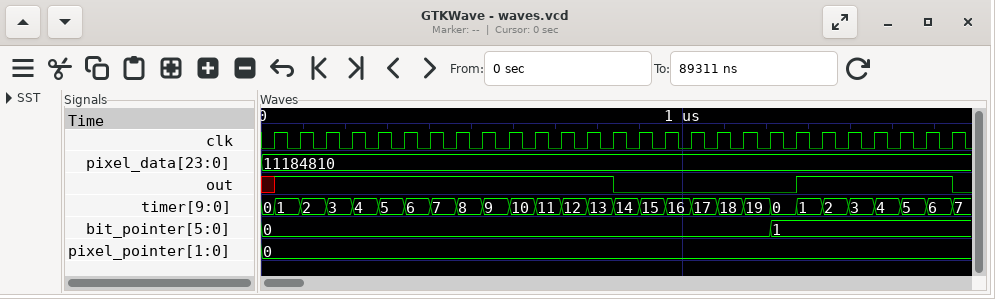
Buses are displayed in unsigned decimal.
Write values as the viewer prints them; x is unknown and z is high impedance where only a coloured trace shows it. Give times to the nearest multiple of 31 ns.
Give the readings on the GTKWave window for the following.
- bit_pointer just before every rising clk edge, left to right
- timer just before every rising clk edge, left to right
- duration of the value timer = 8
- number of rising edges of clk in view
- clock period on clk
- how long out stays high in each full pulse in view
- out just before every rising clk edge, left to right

0, 0, 0, 0, 0, 0, 0, 0, 0, 0, 0, 0, 0, 0, 0, 0, 0, 0, 0, 0, 1, 1, 1, 1, 1, 1, 1
0, 1, 2, 3, 4, 5, 6, 7, 8, 9, 10, 11, 12, 13, 14, 15, 16, 17, 18, 19, 0, 1, 2, 3, 4, 5, 6
62 ns
27
62 ns
372 ns
x 1 1 1 1 1 1 1 1 1 1 1 1 1 0 0 0 0 0 0 0 1 1 1 1 1 1
